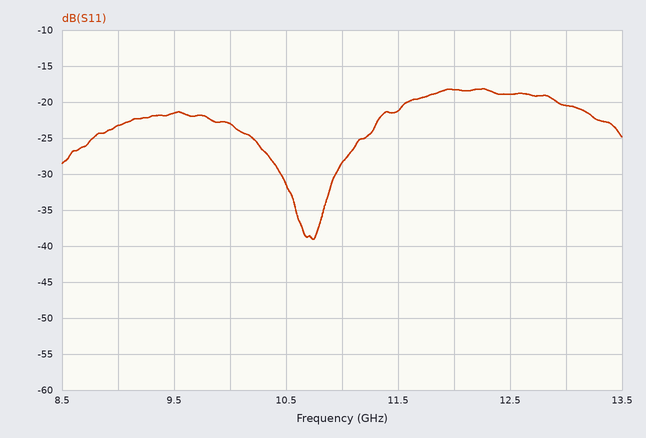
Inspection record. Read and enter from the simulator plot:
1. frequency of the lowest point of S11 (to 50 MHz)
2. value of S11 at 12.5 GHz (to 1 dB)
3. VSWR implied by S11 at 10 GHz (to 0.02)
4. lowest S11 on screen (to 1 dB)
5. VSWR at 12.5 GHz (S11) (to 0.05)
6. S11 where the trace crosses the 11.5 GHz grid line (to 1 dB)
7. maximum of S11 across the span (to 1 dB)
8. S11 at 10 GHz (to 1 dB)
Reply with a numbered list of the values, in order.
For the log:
1. 10.75 GHz
2. -19 dB
3. 1.16
4. -39 dB
5. 1.25
6. -21 dB
7. -18 dB
8. -23 dB
